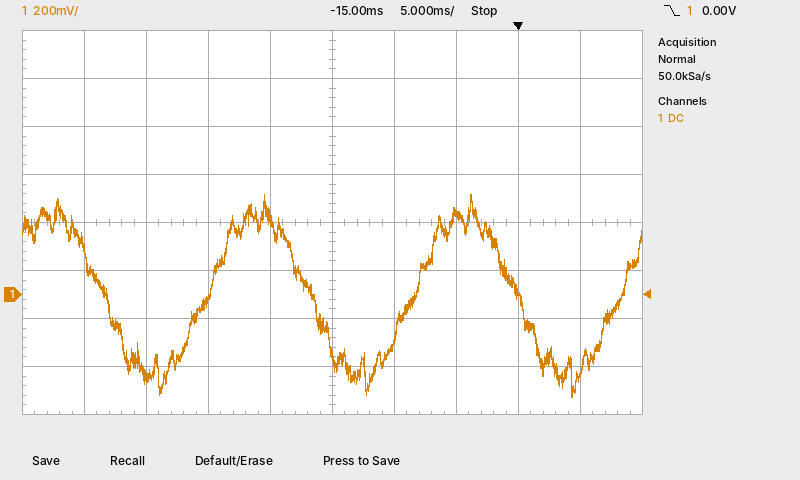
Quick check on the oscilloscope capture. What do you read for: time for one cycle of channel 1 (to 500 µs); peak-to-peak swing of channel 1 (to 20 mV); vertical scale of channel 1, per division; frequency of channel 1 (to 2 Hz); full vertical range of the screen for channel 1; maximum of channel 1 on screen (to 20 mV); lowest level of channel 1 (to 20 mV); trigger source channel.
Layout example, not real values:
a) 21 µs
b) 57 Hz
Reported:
a) 16.5 ms
b) 840 mV
c) 200 mV
d) 60 Hz
e) 1.6 V
f) 420 mV
g) -420 mV
h) channel 1
